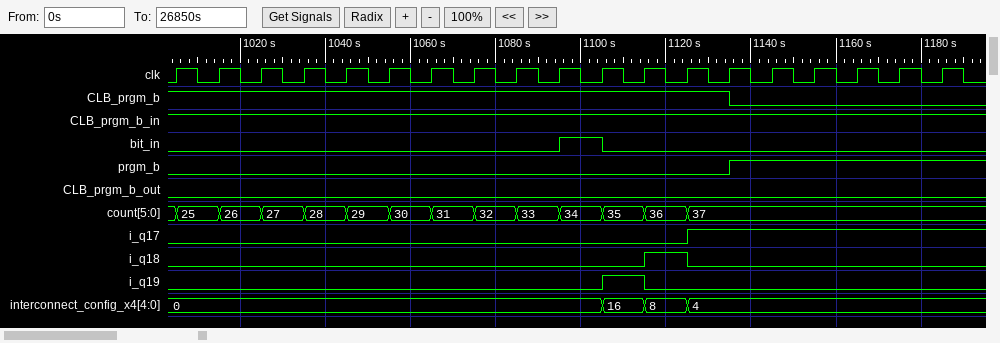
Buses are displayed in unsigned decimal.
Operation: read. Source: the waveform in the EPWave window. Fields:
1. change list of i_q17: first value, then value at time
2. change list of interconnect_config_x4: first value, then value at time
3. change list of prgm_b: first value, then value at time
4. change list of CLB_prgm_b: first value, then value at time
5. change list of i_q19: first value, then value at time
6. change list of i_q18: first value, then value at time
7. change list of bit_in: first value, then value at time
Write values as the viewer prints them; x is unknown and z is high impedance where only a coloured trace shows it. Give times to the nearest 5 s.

0, 1 at 1125 s
0, 16 at 1105 s, 8 at 1115 s, 4 at 1125 s
0, 1 at 1135 s
1, 0 at 1135 s
0, 1 at 1105 s, 0 at 1115 s
0, 1 at 1115 s, 0 at 1125 s
0, 1 at 1095 s, 0 at 1105 s
